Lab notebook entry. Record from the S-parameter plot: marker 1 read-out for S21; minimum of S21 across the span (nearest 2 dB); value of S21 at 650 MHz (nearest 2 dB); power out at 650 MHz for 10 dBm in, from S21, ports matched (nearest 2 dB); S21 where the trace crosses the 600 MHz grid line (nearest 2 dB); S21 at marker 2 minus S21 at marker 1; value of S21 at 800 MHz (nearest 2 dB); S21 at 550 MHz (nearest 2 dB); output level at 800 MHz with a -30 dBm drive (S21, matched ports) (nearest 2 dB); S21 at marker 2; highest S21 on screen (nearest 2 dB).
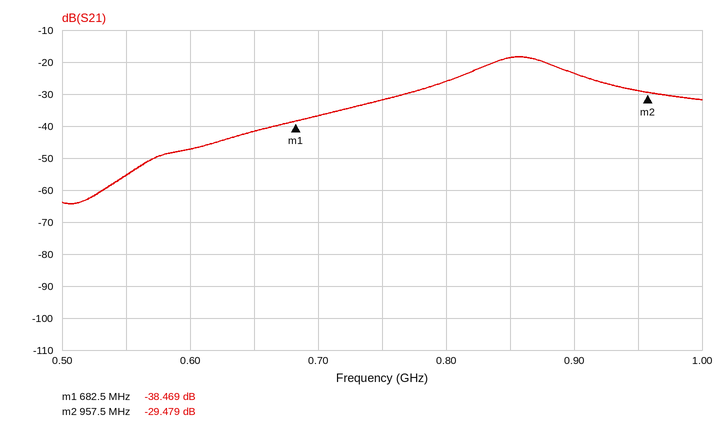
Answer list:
-38.469 dB
-64 dB
-42 dB
-32 dBm
-48 dB
8.990 dB
-26 dB
-56 dB
-56 dBm
-29.479 dB
-18 dB
